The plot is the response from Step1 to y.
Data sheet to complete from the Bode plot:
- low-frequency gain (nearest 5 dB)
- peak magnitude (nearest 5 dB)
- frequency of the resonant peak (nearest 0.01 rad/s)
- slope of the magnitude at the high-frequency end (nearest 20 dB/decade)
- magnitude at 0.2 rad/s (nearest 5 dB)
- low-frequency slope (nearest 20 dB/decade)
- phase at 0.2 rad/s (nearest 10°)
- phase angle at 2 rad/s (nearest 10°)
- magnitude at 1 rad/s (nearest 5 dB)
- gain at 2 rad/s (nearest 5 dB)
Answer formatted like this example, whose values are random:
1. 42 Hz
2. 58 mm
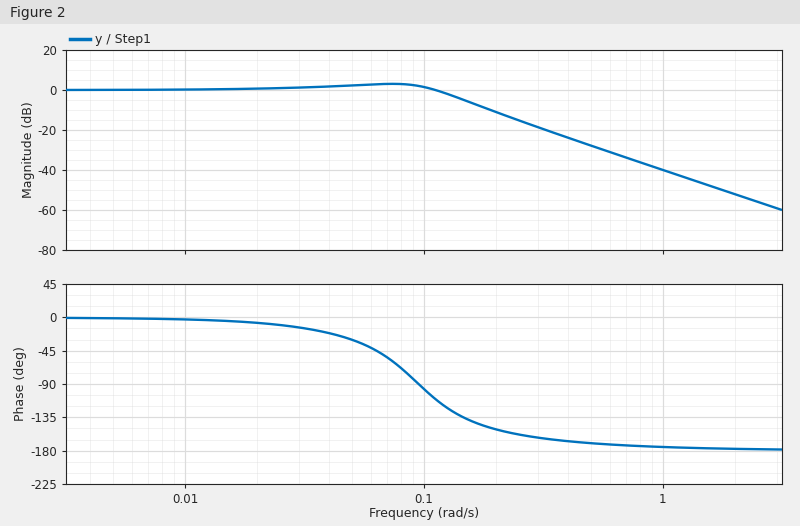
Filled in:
1. 0 dB
2. 5 dB
3. 0.07 rad/s
4. -40 dB/decade
5. -10 dB
6. 0 dB/decade
7. -150°
8. -180°
9. -40 dB
10. -50 dB
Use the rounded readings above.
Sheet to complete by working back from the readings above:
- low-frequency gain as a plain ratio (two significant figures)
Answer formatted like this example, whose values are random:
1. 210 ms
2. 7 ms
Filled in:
1. 1.0
